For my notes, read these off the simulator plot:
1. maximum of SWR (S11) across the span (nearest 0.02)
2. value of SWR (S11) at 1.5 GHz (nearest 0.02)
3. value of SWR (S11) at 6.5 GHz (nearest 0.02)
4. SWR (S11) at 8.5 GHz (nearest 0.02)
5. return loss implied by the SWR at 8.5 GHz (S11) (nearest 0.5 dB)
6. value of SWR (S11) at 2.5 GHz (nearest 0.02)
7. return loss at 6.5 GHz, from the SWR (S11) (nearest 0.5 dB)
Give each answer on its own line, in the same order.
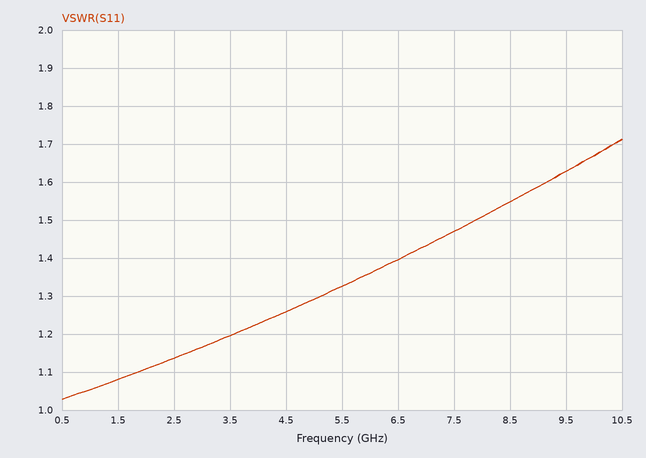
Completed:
1.72
1.08
1.40
1.54
13.5 dB
1.14
15.5 dB
